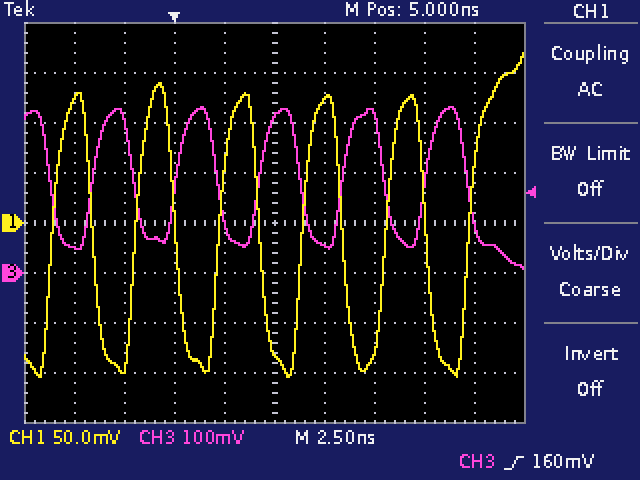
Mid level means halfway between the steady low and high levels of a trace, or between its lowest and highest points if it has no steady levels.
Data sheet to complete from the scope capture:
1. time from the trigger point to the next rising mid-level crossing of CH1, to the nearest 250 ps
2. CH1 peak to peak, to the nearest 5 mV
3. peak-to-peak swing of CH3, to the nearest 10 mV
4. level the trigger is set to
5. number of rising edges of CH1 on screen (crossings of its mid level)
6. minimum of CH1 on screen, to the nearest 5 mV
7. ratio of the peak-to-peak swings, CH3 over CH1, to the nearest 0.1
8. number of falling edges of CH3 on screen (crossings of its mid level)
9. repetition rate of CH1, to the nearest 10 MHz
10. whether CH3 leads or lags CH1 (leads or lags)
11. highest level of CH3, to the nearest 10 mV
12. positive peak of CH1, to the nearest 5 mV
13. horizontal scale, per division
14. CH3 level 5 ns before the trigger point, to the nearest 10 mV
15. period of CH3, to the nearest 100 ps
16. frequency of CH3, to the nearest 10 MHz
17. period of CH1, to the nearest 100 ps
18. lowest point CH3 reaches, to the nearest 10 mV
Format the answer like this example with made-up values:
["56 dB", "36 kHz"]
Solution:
["2.25 ns", "325 mV", "320 mV", "160 mV", "6", "-155 mV", "1.0", "6", "240 MHz", "lags", "330 mV", "170 mV", "2.5 ns", "50 mV", "4.2 ns", "240 MHz", "4.2 ns", "10 mV"]
